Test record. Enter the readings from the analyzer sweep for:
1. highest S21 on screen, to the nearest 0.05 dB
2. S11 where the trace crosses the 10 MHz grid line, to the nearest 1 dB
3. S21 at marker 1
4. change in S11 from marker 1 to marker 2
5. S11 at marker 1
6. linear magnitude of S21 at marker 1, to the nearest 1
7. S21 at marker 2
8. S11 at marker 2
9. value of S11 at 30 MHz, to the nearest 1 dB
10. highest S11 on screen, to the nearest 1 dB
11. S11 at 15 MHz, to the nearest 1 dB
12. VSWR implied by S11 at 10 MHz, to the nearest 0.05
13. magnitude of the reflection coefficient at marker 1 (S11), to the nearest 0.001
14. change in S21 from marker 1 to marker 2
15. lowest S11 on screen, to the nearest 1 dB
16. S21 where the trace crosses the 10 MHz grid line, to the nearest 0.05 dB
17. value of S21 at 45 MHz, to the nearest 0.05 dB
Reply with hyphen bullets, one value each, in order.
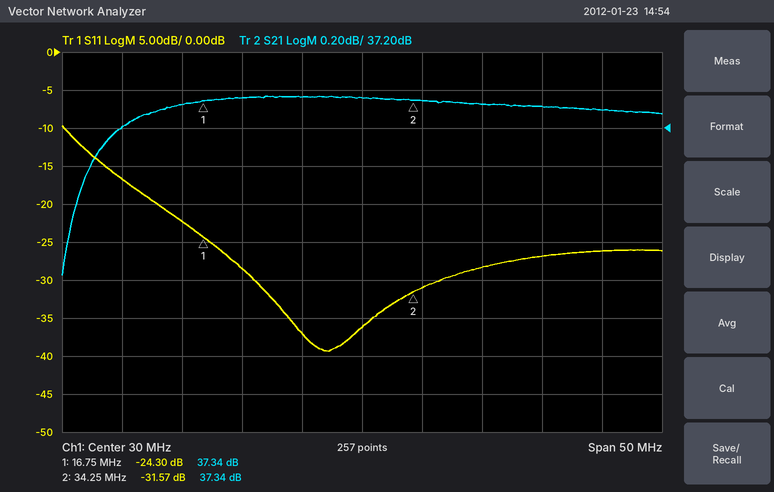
- 37.35 dB
- -17 dB
- 37.34 dB
- -7.27 dB
- -24.30 dB
- 74
- 37.34 dB
- -31.57 dB
- -36 dB
- -10 dB
- -22 dB
- 1.35
- 0.061
- 0.00 dB
- -39 dB
- 37.20 dB
- 37.30 dB
